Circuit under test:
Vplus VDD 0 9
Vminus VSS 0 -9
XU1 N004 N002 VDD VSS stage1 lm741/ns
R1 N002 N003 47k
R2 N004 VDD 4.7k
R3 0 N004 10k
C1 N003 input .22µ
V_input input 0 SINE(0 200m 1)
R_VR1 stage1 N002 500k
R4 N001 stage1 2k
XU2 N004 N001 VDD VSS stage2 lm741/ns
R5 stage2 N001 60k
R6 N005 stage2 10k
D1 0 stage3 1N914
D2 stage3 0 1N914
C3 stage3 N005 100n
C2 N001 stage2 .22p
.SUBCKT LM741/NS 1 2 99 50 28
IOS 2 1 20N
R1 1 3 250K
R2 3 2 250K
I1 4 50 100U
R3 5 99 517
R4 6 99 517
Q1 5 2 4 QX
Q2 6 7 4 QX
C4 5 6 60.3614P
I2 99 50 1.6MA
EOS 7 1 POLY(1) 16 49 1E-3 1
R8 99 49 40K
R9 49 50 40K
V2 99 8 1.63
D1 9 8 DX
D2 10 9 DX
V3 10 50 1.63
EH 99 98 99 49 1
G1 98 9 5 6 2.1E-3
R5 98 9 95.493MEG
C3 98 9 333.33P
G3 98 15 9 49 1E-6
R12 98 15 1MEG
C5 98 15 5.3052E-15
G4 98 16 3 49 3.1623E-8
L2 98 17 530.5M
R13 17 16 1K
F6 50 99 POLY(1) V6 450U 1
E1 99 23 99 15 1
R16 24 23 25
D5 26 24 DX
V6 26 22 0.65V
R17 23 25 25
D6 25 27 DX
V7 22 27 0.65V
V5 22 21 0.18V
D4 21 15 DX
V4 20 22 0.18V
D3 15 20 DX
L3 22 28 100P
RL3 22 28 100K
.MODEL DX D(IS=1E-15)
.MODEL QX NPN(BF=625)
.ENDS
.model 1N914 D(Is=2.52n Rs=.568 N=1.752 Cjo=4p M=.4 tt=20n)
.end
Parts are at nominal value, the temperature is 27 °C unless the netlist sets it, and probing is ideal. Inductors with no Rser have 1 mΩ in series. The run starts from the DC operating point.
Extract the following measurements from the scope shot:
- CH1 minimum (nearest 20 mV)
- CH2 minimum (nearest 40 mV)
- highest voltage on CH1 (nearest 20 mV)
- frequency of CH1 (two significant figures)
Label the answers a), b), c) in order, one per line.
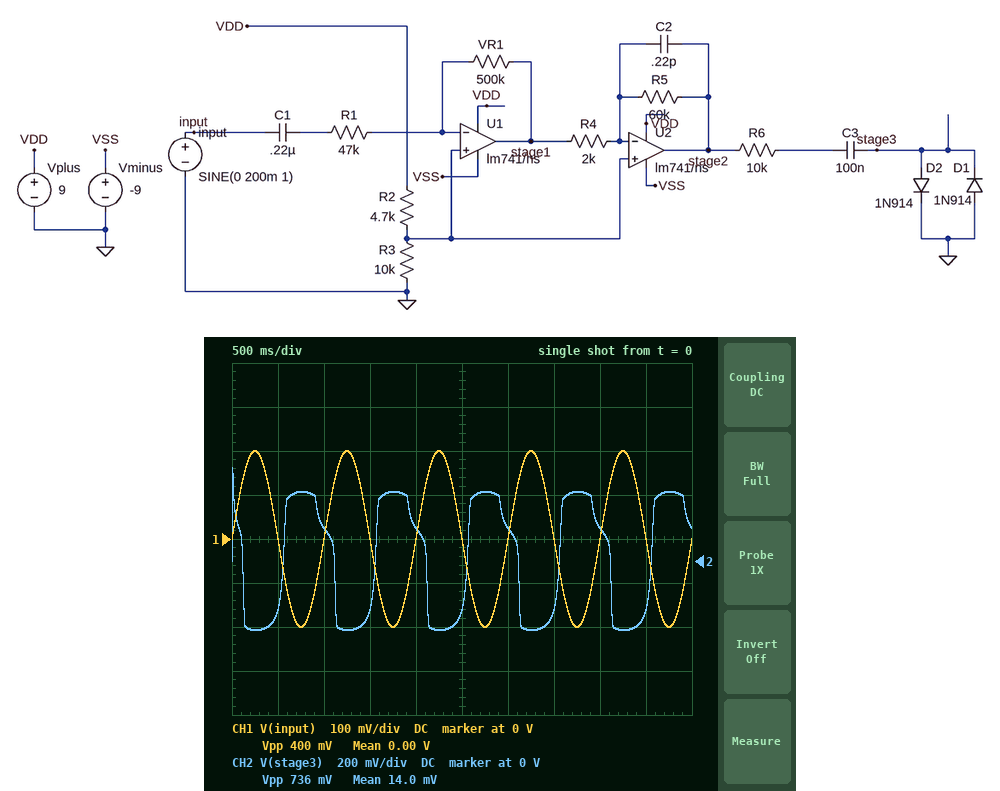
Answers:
a) -200 mV
b) -320 mV
c) 200 mV
d) 1.0 Hz
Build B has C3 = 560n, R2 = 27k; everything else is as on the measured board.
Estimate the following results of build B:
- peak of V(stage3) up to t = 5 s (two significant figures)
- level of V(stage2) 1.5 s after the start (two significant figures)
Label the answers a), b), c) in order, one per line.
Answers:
a) 480 mV
b) -3.2 V
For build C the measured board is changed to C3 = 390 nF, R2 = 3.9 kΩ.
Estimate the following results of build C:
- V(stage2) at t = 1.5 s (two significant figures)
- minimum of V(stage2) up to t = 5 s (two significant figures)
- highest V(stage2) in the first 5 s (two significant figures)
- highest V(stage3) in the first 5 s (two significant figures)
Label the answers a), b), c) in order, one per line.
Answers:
a) 820 mV
b) 810 mV
c) 8.0 V
d) 470 mV
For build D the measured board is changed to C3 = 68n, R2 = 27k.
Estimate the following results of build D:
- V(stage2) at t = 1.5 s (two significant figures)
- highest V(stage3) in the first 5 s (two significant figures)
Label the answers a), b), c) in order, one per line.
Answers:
a) -3.2 V
b) 410 mV
